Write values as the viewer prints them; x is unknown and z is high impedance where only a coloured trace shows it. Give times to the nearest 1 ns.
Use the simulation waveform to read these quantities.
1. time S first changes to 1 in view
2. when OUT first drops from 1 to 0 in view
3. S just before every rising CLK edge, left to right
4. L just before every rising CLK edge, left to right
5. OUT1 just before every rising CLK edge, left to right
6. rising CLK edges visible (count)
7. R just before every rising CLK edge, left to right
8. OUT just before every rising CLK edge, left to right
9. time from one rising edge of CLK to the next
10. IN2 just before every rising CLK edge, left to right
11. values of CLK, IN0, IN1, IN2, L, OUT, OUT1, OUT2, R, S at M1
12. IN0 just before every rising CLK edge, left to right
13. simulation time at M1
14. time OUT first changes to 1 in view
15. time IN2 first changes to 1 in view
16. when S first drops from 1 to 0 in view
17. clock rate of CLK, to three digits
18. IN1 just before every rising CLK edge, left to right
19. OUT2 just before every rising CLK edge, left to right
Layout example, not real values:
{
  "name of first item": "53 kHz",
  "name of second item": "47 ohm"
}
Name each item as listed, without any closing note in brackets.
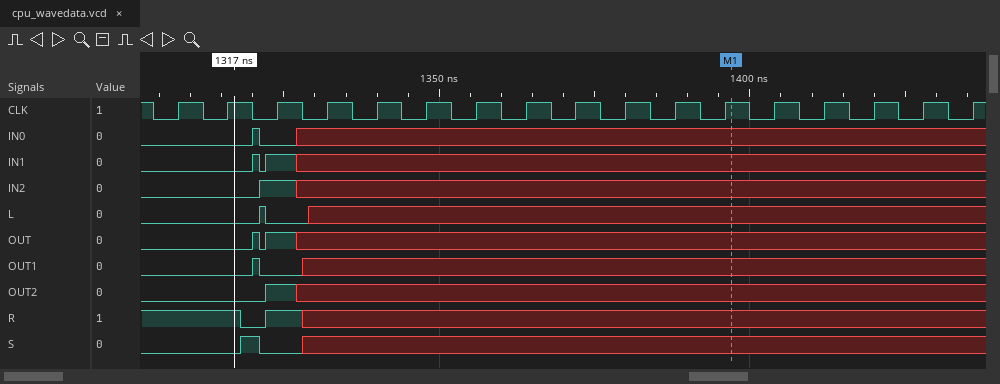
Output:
{
  "time S first changes to 1 in view": "1318 ns",
  "when OUT first drops from 1 to 0 in view": "1321 ns",
  "S just before every rising CLK edge, left to right": "0 0 0 x x x x x x x x x x x x x x",
  "L just before every rising CLK edge, left to right": "0 0 0 x x x x x x x x x x x x x x",
  "OUT1 just before every rising CLK edge, left to right": "0 0 0 x x x x x x x x x x x x x x",
  "rising CLK edges visible": "17",
  "R just before every rising CLK edge, left to right": "1 1 1 x x x x x x x x x x x x x x",
  "OUT just before every rising CLK edge, left to right": "0 0 1 x x x x x x x x x x x x x x",
  "time from one rising edge of CLK to the next": "8 ns",
  "IN2 just before every rising CLK edge, left to right": "0 0 1 x x x x x x x x x x x x x x",
  "values of CLK, IN0, IN1, IN2, L, OUT, OUT1, OUT2, R, S at M1": "CLK=1, IN0=x, IN1=x, IN2=x, L=x, OUT=x, OUT1=x, OUT2=x, R=x, S=x",
  "IN0 just before every rising CLK edge, left to right": "0 0 0 x x x x x x x x x x x x x x",
  "simulation time at M1": "1397 ns",
  "time OUT first changes to 1 in view": "1320 ns",
  "time IN2 first changes to 1 in view": "1321 ns",
  "when S first drops from 1 to 0 in view": "1321 ns",
  "clock rate of CLK, to three digits": "125 MHz",
  "IN1 just before every rising CLK edge, left to right": "0 0 1 x x x x x x x x x x x x x x",
  "OUT2 just before every rising CLK edge, left to right": "0 0 1 x x x x x x x x x x x x x x"
}
